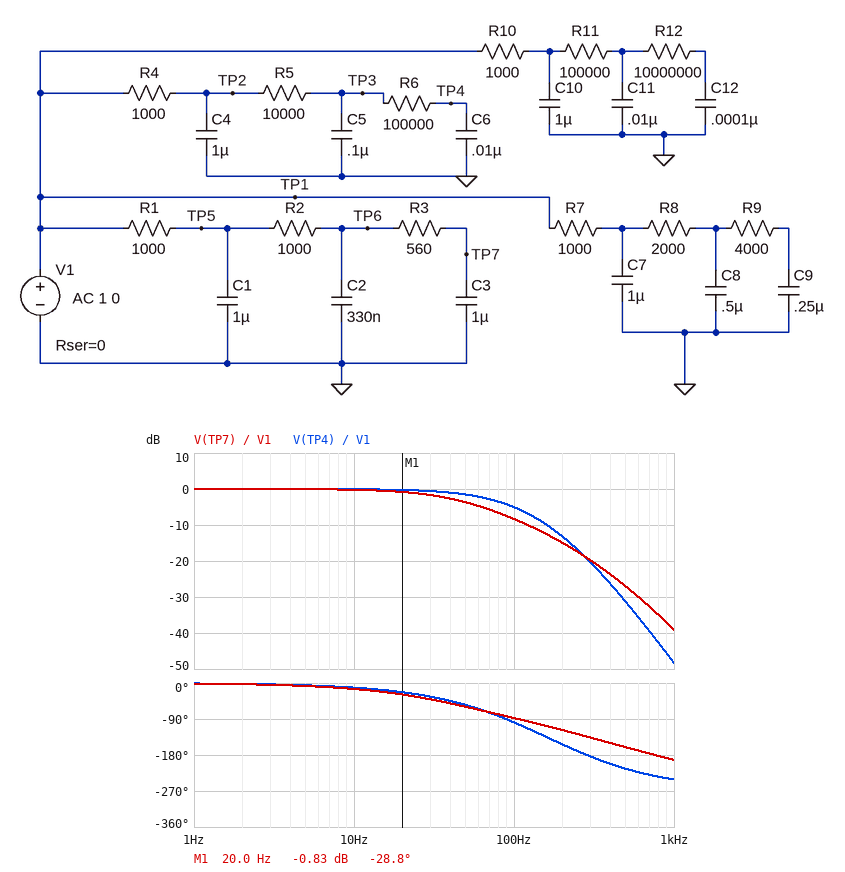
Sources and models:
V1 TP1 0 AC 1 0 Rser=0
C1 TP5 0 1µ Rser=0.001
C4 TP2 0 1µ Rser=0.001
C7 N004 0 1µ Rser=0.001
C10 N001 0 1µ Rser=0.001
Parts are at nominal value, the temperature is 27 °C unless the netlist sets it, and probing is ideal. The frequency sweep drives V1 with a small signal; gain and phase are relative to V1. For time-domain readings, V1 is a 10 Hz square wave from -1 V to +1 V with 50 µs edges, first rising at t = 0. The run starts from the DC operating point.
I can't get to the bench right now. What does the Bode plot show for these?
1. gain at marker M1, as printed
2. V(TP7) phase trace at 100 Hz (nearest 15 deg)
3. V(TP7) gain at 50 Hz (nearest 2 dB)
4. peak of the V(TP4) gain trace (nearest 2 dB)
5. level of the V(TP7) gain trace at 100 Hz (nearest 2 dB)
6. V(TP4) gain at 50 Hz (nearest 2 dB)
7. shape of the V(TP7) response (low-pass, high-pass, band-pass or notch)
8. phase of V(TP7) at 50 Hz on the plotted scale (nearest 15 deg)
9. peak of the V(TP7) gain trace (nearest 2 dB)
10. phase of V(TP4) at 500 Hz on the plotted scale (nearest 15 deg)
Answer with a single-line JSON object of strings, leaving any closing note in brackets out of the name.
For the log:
{"gain at marker M1, as printed": "-0.83 dB", "V(TP7) phase trace at 100 Hz": "-90 deg", "V(TP7) gain at 50 Hz": "-4 dB", "peak of the V(TP4) gain trace": "0 dB", "level of the V(TP7) gain trace at 100 Hz": "-8 dB", "V(TP4) gain at 50 Hz": "-2 dB", "shape of the V(TP7) response": "low-pass", "phase of V(TP7) at 50 Hz on the plotted scale": "-60 deg", "peak of the V(TP7) gain trace": "0 dB", "phase of V(TP4) at 500 Hz on the plotted scale": "-210 deg"}
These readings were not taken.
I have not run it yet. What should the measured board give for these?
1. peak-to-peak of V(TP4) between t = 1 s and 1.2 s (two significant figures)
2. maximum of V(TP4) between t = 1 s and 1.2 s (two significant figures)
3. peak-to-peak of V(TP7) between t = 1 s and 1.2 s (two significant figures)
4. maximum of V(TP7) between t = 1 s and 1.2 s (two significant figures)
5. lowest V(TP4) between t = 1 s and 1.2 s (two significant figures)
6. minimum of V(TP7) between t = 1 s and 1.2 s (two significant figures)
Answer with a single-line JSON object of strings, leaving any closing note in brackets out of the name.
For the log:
{"peak-to-peak of V(TP4) between t = 1 s and 1.2 s": "2.0 V", "maximum of V(TP4) between t = 1 s and 1.2 s": "1.0 V", "peak-to-peak of V(TP7) between t = 1 s and 1.2 s": "2.0 V", "maximum of V(TP7) between t = 1 s and 1.2 s": "1.0 V", "lowest V(TP4) between t = 1 s and 1.2 s": "-1.0 V", "minimum of V(TP7) between t = 1 s and 1.2 s": "-1.0 V"}
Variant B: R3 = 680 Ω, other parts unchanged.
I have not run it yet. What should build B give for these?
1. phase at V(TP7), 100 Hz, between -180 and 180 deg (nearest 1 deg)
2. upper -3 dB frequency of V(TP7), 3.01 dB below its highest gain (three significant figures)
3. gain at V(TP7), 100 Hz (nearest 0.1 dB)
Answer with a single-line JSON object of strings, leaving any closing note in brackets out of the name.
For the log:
{"phase at V(TP7), 100 Hz, between -180 and 180 deg": "-89 deg", "upper -3 dB frequency of V(TP7), 3.01 dB below its highest gain": "42.2 Hz", "gain at V(TP7), 100 Hz": "-8.5 dB"}
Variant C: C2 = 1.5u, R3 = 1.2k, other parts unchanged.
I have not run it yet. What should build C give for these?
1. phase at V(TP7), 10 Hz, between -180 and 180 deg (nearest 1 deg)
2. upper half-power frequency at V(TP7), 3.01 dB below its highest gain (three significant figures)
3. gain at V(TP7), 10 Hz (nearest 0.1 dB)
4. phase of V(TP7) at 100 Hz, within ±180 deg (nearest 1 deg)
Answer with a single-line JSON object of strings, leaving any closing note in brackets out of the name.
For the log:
{"phase at V(TP7), 10 Hz, between -180 and 180 deg": "-25 deg", "upper half-power frequency at V(TP7), 3.01 dB below its highest gain": "25.8 Hz", "gain at V(TP7), 10 Hz": "-0.6 dB", "phase of V(TP7) at 100 Hz, within ±180 deg": "-115 deg"}
